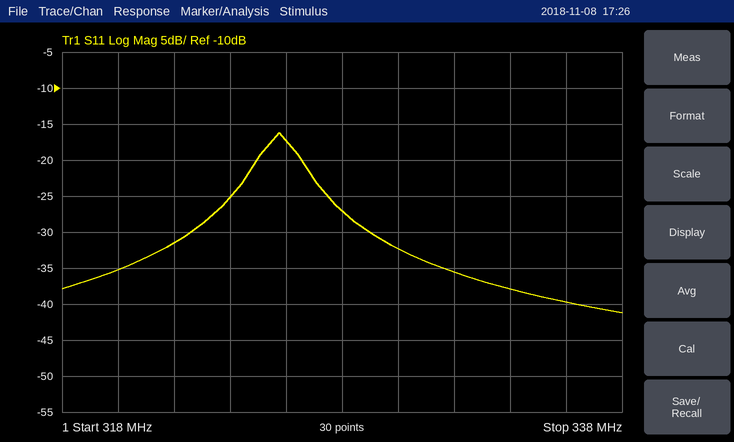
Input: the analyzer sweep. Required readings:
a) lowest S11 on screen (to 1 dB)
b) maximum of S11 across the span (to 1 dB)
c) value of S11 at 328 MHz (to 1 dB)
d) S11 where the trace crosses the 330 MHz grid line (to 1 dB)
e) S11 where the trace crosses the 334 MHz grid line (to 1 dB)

-41 dB
-16 dB
-27 dB
-32 dB
-38 dB
